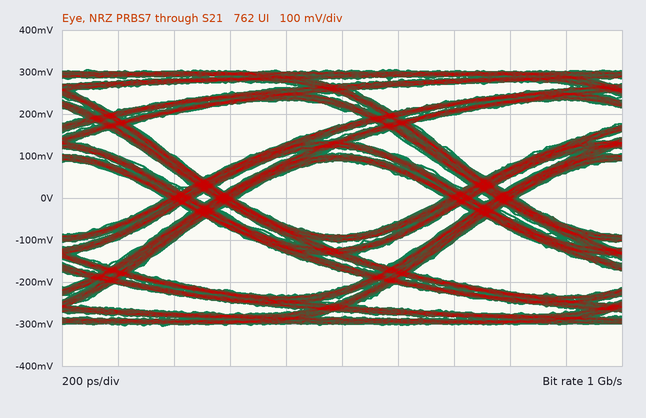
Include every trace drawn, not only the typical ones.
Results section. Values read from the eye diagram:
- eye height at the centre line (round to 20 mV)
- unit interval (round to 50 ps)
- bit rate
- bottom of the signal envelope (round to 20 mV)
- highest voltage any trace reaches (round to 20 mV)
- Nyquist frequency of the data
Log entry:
180 mV
1.00 ns
1 Gb/s
-300 mV
300 mV
500 MHz
